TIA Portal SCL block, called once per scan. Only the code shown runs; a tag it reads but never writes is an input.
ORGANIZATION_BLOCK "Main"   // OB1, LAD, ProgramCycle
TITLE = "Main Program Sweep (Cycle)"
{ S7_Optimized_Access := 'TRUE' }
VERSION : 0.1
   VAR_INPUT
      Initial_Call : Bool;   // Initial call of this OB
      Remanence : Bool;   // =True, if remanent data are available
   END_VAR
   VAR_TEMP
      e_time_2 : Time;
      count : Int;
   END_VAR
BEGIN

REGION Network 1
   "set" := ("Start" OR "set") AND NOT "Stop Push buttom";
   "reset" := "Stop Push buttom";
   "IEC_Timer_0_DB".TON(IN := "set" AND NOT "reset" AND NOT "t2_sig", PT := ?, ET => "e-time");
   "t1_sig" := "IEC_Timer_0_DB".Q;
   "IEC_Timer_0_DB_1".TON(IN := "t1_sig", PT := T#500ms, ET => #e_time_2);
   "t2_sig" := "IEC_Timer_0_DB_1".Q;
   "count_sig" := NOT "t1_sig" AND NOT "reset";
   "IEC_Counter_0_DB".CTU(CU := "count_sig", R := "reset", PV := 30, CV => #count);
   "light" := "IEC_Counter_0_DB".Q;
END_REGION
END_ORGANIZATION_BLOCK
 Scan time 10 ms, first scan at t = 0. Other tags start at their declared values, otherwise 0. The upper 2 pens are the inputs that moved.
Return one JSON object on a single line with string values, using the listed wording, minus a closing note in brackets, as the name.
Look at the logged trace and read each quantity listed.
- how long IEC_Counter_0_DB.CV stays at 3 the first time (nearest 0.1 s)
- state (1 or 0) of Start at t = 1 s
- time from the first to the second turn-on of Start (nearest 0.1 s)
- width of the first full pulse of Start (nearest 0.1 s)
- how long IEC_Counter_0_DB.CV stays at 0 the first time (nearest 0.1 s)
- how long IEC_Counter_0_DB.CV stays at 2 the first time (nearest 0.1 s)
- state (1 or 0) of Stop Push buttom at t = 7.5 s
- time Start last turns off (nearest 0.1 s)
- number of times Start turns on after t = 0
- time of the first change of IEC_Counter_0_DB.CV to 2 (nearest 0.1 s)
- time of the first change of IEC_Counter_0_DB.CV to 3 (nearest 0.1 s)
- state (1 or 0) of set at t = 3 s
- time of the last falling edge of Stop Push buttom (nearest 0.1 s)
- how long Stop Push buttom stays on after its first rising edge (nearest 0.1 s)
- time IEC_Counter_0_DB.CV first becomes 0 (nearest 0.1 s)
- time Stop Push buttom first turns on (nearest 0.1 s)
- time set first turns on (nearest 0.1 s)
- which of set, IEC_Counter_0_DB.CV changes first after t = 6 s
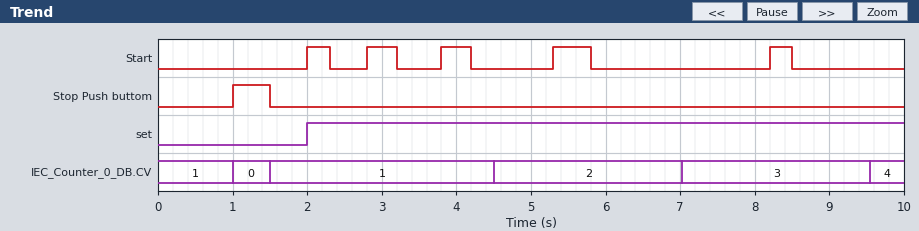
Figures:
{"how long IEC_Counter_0_DB.CV stays at 3 the first time": "2.5 s", "state (1 or 0) of Start at t = 1 s": "0", "time from the first to the second turn-on of Start": "0.8 s", "width of the first full pulse of Start": "0.3 s", "how long IEC_Counter_0_DB.CV stays at 0 the first time": "0.5 s", "how long IEC_Counter_0_DB.CV stays at 2 the first time": "2.5 s", "state (1 or 0) of Stop Push buttom at t = 7.5 s": "0", "time Start last turns off": "8.5 s", "number of times Start turns on after t = 0": "5", "time of the first change of IEC_Counter_0_DB.CV to 2": "4.5 s", "time of the first change of IEC_Counter_0_DB.CV to 3": "7.0 s", "state (1 or 0) of set at t = 3 s": "1", "time of the last falling edge of Stop Push buttom": "1.5 s", "how long Stop Push buttom stays on after its first rising edge": "0.5 s", "time IEC_Counter_0_DB.CV first becomes 0": "1.0 s", "time Stop Push buttom first turns on": "1.0 s", "time set first turns on": "2.0 s", "which of set, IEC_Counter_0_DB.CV changes first after t = 6 s": "IEC_Counter_0_DB.CV"}
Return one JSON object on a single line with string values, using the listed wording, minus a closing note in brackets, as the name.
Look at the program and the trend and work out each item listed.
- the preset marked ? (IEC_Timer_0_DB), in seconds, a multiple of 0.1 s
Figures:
{"the preset marked ? (IEC_Timer_0_DB), in seconds, a multiple of 0.1 s": "2.0 s"}
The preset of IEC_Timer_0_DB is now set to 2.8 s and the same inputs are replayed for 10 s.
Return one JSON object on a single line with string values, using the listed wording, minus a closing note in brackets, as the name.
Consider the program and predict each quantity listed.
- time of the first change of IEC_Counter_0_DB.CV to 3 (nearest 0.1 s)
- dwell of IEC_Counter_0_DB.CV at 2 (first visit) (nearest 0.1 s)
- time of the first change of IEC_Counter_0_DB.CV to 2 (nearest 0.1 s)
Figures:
{"time of the first change of IEC_Counter_0_DB.CV to 3": "8.6 s", "dwell of IEC_Counter_0_DB.CV at 2 (first visit)": "3.3 s", "time of the first change of IEC_Counter_0_DB.CV to 2": "5.3 s"}
